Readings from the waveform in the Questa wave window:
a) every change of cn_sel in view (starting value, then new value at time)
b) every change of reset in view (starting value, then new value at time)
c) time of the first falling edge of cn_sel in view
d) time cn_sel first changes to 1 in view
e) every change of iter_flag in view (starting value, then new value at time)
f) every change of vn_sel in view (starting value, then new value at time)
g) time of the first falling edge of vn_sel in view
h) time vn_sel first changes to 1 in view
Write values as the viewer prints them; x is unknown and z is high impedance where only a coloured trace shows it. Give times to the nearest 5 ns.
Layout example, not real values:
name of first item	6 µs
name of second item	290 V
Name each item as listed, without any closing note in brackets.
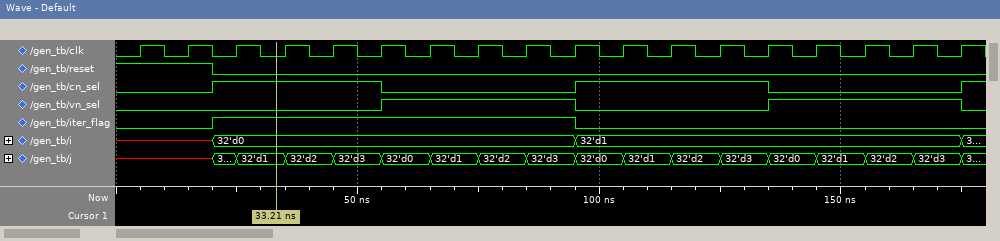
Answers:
every change of cn_sel in view	0, 1 at 20 ns, 0 at 55 ns, 1 at 95 ns, 0 at 135 ns, 1 at 175 ns
every change of reset in view	1, 0 at 20 ns
time of the first falling edge of cn_sel in view	55 ns
time cn_sel first changes to 1 in view	20 ns
every change of iter_flag in view	0, 1 at 20 ns, 0 at 95 ns
every change of vn_sel in view	0, 1 at 55 ns, 0 at 95 ns, 1 at 135 ns, 0 at 175 ns
time of the first falling edge of vn_sel in view	95 ns
time vn_sel first changes to 1 in view	55 ns
